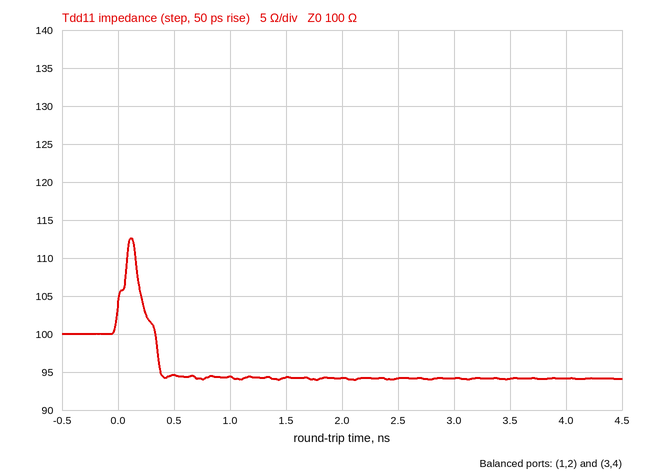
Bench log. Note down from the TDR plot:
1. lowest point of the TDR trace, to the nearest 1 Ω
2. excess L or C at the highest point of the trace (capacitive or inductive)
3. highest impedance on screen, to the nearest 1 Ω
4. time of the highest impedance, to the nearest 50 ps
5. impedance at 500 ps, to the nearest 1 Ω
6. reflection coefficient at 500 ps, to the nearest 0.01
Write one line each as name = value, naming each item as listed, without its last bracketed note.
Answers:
lowest point of the TDR trace, to the nearest 1 Ω = 94 Ω
excess L or C at the highest point of the trace = inductive
highest impedance on screen, to the nearest 1 Ω = 113 Ω
time of the highest impedance, to the nearest 50 ps = 100 ps
impedance at 500 ps, to the nearest 1 Ω = 95 Ω
reflection coefficient at 500 ps, to the nearest 0.01 = -0.03
